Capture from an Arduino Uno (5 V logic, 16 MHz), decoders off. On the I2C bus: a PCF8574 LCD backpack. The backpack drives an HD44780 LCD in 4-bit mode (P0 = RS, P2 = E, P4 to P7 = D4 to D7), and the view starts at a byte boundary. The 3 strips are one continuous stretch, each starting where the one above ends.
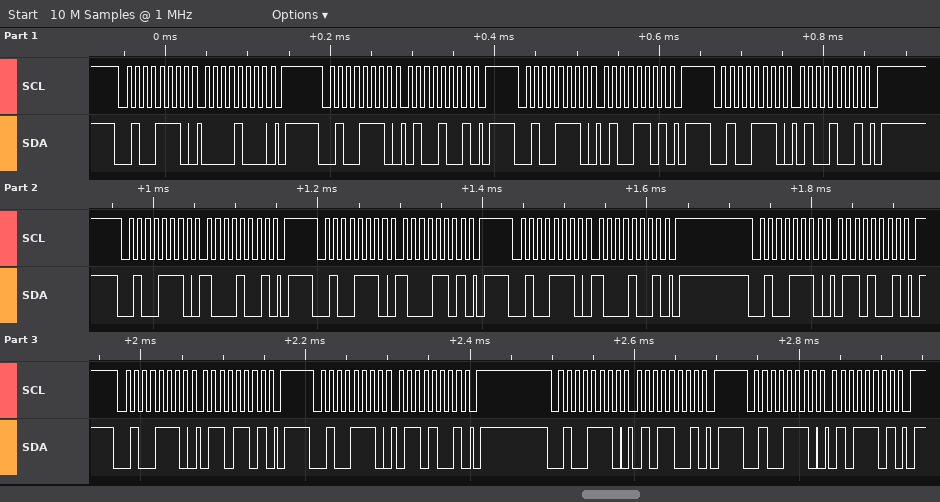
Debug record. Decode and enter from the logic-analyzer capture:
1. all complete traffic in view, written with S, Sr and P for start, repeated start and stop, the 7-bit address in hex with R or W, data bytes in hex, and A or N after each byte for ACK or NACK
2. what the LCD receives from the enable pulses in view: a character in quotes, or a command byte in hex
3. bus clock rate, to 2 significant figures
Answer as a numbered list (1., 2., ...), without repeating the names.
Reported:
1. S 27W A 08 A P S 27W A 49 A P S 27W A 4D A P S 27W A 49 A P S 27W A 89 A P S 27W A 8D A P S 27W A 89 A P S 27W A 69 A P S 27W A 6D A P S 27W A 69 A P S 27W A 59 A P S 27W A 5D A P
2. 'H'
3. 100 kHz
